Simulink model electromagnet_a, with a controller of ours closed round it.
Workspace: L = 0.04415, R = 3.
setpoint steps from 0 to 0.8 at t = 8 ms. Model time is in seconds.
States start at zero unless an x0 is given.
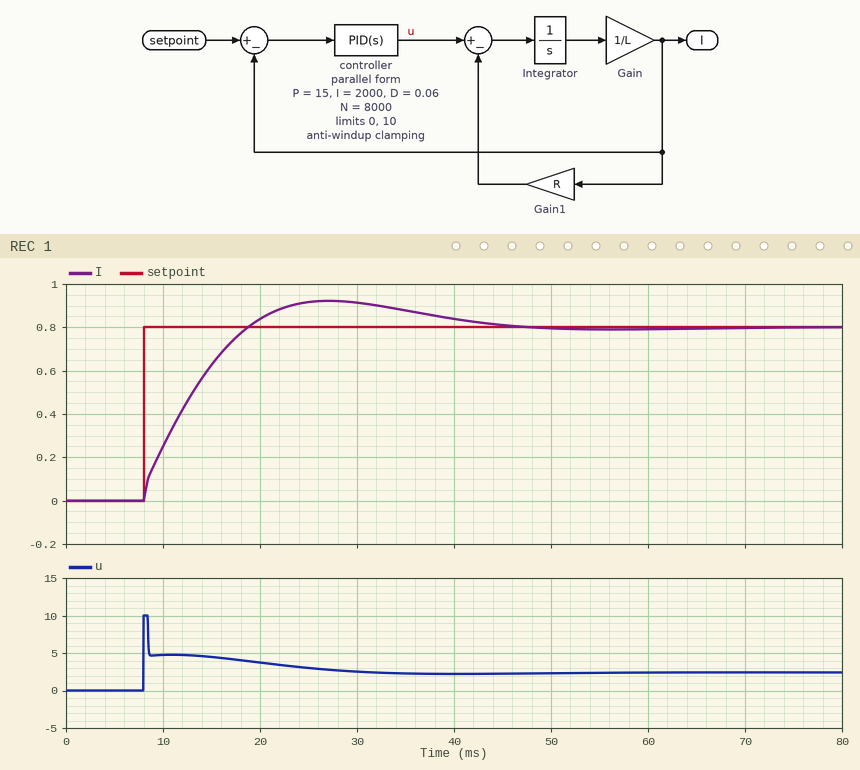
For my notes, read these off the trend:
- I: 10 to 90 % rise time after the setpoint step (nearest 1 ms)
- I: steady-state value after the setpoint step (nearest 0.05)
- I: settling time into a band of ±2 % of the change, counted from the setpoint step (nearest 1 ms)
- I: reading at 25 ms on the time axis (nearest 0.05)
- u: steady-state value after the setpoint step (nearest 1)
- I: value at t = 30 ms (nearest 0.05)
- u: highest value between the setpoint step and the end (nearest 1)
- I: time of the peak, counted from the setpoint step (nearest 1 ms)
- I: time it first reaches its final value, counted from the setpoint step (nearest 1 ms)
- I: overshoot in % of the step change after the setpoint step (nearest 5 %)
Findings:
8 ms
0.80
36 ms
0.90
2
0.90
10
19 ms
11 ms
15 %
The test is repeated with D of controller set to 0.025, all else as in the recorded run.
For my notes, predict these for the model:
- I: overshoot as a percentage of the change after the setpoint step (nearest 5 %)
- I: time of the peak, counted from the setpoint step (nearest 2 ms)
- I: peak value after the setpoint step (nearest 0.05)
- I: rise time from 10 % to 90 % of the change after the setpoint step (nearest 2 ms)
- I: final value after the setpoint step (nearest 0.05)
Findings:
10 %
16 ms
0.90
6 ms
0.80
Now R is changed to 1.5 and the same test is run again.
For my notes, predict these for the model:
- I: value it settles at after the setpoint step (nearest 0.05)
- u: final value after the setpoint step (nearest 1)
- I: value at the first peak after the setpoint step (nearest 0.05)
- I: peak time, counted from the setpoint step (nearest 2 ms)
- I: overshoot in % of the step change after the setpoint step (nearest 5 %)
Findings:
0.80
1
0.95
18 ms
20 %
